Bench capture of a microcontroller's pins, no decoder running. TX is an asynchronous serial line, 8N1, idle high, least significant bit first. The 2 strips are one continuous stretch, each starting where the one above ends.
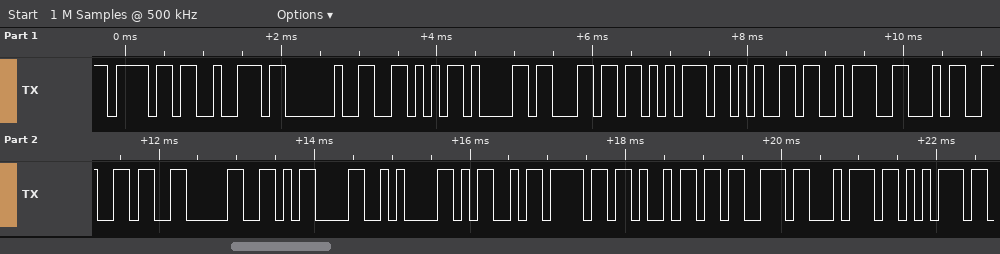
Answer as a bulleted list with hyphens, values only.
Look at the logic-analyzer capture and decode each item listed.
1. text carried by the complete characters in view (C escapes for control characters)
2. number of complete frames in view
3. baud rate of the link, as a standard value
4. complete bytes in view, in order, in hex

- "or Value:460\r\nMoistu"
- 20
- 9600 baud
- 6F 72 20 56 61 6C 75 65 3A 34 36 30 0D 0A 4D 6F 69 73 74 75
